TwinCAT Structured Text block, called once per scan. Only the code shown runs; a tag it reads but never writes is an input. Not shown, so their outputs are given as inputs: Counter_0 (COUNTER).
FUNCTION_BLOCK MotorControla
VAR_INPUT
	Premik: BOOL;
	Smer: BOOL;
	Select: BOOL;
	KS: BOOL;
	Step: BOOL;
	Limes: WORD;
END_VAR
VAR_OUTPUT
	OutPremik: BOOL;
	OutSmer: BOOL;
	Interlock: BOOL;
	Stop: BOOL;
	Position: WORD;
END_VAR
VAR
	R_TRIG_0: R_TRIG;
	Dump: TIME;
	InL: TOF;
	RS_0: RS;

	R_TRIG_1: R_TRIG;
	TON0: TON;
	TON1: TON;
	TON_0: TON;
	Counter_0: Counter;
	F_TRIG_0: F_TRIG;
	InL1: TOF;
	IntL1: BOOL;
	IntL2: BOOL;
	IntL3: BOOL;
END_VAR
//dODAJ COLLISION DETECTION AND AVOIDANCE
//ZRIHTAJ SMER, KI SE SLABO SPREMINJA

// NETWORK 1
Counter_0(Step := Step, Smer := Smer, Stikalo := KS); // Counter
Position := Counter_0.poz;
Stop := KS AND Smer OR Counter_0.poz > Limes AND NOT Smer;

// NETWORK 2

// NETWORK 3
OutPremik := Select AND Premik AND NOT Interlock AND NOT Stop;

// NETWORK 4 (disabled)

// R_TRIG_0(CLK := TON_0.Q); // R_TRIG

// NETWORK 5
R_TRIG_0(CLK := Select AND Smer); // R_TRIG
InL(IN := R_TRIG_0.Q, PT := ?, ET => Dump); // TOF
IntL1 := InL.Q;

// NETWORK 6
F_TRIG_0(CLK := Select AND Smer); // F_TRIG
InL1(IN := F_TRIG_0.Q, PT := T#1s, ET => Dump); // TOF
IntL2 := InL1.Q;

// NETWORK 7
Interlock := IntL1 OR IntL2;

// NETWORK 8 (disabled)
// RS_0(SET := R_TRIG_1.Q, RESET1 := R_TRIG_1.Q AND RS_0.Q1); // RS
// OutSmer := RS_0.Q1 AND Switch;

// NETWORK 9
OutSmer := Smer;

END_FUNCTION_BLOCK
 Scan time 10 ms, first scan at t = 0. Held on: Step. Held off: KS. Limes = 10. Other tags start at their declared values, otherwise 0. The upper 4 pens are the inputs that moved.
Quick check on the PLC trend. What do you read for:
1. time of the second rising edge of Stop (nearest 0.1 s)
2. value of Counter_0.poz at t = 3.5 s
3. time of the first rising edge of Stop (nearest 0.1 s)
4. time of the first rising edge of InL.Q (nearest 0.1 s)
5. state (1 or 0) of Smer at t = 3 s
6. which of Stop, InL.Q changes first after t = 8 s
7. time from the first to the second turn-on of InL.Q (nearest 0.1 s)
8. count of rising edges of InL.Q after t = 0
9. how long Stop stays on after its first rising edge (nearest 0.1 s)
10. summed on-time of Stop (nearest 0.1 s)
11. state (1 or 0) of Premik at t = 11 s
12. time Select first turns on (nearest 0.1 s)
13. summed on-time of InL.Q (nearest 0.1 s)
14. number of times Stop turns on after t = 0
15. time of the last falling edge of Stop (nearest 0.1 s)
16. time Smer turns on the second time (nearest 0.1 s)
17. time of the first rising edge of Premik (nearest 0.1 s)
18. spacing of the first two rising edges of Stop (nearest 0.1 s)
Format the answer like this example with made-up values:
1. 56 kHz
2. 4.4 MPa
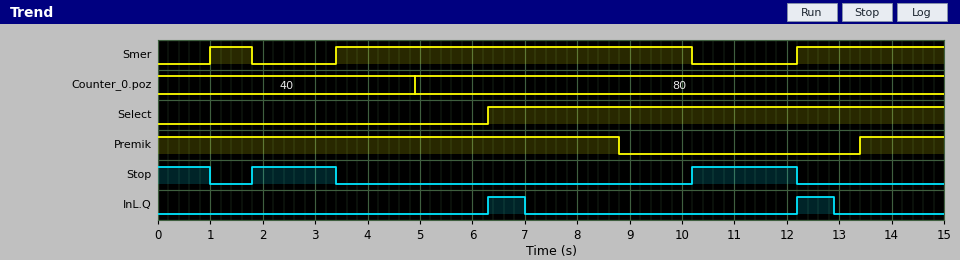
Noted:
1. 10.2 s
2. 40
3. 1.8 s
4. 6.3 s
5. 0
6. Stop
7. 5.9 s
8. 2
9. 1.6 s
10. 4.6 s
11. 0
12. 6.3 s
13. 1.4 s
14. 2
15. 12.2 s
16. 3.4 s
17. 13.4 s
18. 8.4 s
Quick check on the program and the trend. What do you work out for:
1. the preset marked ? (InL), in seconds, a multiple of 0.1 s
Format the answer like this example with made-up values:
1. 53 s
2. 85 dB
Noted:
1. 0.7 s
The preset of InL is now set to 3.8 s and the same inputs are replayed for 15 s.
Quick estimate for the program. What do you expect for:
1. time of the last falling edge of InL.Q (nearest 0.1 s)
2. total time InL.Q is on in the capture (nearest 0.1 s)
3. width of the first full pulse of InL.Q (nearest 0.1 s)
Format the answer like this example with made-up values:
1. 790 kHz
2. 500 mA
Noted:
1. 10.1 s
2. 6.6 s
3. 3.8 s
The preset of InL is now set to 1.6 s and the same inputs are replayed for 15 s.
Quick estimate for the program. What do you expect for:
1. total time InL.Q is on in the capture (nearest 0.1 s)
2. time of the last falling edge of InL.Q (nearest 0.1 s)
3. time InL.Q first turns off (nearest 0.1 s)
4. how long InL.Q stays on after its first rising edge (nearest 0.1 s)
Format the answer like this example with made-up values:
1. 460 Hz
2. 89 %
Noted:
1. 3.2 s
2. 13.8 s
3. 7.9 s
4. 1.6 s
